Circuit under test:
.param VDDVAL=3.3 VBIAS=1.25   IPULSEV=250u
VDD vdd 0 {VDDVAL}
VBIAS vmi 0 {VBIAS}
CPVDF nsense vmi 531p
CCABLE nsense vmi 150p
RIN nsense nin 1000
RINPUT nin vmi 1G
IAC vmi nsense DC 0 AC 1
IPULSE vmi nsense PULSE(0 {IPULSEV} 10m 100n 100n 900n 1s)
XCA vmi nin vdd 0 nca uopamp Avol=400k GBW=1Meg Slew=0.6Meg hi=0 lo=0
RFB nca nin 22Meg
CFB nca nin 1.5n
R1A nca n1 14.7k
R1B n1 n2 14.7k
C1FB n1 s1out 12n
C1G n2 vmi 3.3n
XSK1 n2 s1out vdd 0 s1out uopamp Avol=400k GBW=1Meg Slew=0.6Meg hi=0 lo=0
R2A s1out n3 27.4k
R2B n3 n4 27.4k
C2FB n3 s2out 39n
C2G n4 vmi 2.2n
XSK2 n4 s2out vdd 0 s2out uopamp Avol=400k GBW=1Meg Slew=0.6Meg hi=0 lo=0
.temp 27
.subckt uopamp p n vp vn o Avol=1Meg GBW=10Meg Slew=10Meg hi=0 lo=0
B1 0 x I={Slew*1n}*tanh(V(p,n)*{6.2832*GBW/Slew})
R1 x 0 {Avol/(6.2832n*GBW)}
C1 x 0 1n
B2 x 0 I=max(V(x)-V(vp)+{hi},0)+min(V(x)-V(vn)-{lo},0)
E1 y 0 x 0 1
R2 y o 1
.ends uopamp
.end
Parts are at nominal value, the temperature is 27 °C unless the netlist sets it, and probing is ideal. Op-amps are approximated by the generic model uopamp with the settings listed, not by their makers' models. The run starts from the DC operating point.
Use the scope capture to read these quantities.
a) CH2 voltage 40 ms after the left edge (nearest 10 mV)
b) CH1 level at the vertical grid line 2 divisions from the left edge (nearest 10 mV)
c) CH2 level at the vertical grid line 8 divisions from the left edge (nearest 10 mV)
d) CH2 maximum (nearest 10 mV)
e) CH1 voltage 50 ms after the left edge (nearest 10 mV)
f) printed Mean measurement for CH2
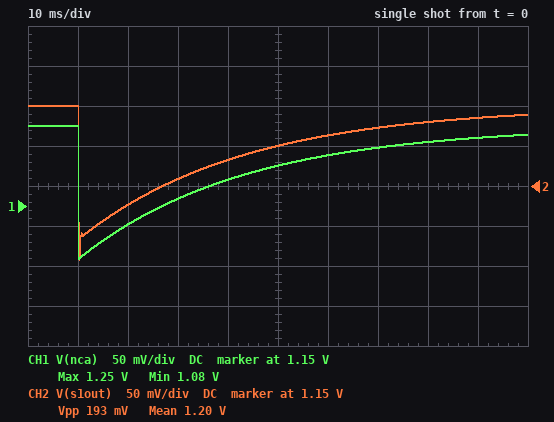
1.18 V
1.13 V
1.23 V
1.25 V
1.20 V
1.20 V
